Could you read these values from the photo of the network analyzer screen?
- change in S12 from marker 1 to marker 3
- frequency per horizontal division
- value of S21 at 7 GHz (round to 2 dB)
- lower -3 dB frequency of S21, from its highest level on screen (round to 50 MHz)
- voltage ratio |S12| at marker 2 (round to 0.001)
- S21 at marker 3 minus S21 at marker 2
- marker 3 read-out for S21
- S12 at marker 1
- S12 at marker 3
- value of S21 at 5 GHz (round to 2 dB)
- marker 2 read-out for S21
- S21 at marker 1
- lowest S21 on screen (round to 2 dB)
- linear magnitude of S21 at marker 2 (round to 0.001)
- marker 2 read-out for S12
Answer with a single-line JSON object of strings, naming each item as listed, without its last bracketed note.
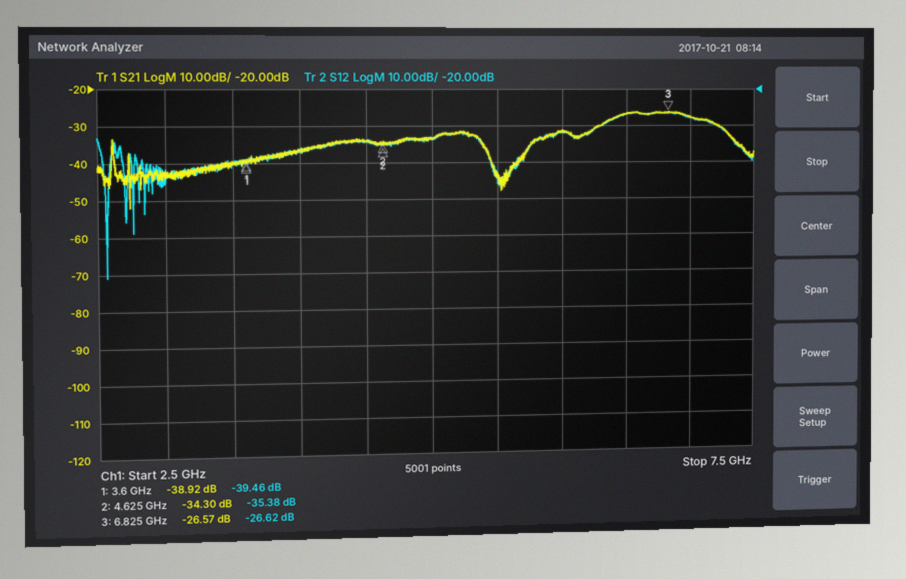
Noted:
{"change in S12 from marker 1 to marker 3": "12.84 dB", "frequency per horizontal division": "500 MHz", "value of S21 at 7 GHz": "-28 dB", "lower -3 dB frequency of S21, from its highest level on screen": "6.35 GHz", "voltage ratio |S12| at marker 2": "0.017", "S21 at marker 3 minus S21 at marker 2": "7.73 dB", "marker 3 read-out for S21": "-26.57 dB", "S12 at marker 1": "-39.46 dB", "S12 at marker 3": "-26.62 dB", "value of S21 at 5 GHz": "-34 dB", "marker 2 read-out for S21": "-34.30 dB", "S21 at marker 1": "-38.92 dB", "lowest S21 on screen": "-52 dB", "linear magnitude of S21 at marker 2": "0.019", "marker 2 read-out for S12": "-35.38 dB"}
